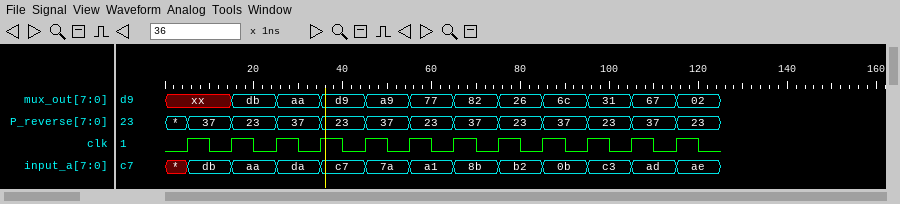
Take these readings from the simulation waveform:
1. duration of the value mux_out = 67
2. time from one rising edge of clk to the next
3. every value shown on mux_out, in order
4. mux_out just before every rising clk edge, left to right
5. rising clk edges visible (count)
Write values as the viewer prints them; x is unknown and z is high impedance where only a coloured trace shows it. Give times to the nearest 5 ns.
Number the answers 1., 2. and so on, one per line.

1. 10 ns
2. 10 ns
3. xx, db, aa, d9, a9, 77, 82, 26, 6c, 31, 67, 02
4. xx, xx, db, aa, d9, a9, 77, 82, 26, 6c, 31, 67
5. 12
